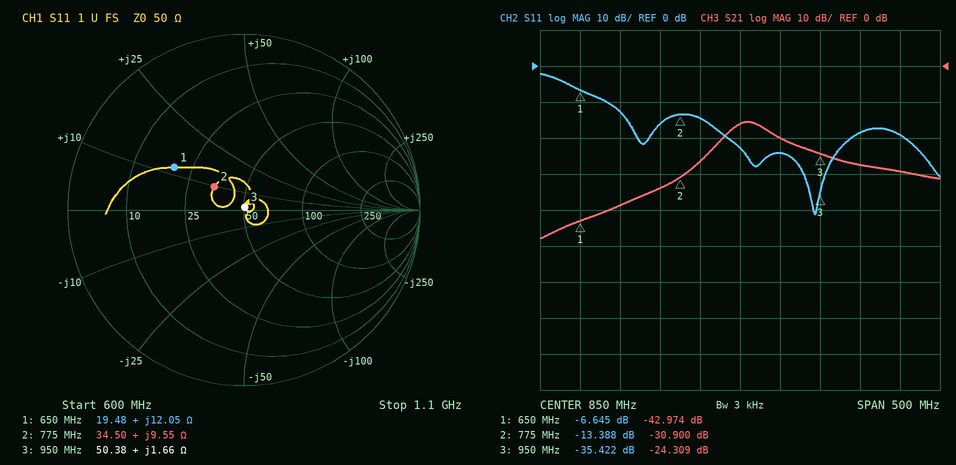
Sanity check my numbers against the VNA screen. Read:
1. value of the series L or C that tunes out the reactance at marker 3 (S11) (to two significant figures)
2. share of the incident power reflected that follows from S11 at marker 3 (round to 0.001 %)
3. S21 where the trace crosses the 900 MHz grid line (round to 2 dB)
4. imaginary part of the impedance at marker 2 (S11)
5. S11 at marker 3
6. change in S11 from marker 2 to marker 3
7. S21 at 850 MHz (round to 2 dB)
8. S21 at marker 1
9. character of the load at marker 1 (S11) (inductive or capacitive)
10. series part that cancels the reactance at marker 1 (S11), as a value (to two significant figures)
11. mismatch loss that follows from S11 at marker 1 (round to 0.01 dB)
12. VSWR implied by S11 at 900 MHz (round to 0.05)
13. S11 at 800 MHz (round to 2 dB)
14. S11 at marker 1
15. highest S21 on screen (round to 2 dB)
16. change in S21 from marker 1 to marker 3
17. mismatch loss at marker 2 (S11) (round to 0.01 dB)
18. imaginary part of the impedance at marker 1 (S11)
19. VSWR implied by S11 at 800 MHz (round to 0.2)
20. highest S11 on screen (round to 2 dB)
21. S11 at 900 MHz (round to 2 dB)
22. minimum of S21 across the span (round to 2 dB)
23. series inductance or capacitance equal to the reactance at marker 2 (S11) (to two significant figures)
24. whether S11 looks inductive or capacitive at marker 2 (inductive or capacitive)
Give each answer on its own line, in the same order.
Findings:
100 pF
0.029 %
-20 dB
+9.55 Ω
-35.422 dB
-22.034 dB
-16 dB
-42.974 dB
inductive
20 pF
1.06 dB
1.15
-14 dB
-6.645 dB
-16 dB
18.665 dB
0.20 dB
+12.05 Ω
1.4
-2 dB
-24 dB
-48 dB
2.0 nH
inductive
